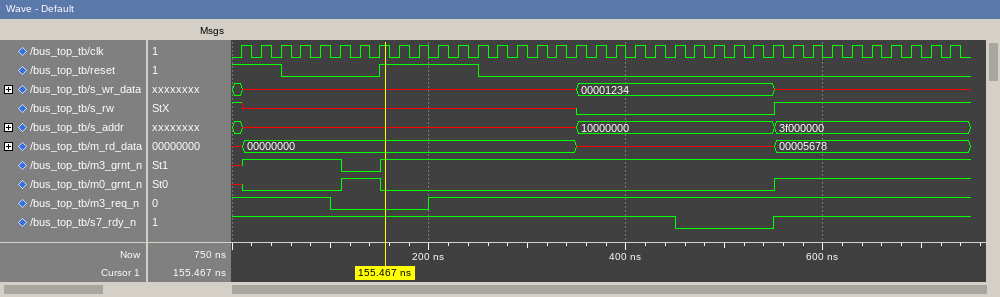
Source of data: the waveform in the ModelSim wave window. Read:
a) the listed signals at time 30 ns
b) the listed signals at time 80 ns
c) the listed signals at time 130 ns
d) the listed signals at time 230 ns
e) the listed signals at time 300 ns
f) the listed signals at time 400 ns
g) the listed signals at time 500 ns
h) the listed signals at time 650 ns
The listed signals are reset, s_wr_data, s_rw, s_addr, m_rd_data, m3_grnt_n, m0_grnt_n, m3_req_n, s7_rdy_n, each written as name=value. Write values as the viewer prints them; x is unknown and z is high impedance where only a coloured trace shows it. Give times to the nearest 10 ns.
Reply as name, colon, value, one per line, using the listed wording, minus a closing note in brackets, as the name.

the listed signals at time 30 ns: reset=1, s_wr_data=x, s_rw=x, s_addr=x, m_rd_data=00000000, m3_grnt_n=1, m0_grnt_n=0, m3_req_n=1, s7_rdy_n=1
the listed signals at time 80 ns: reset=0, s_wr_data=x, s_rw=x, s_addr=x, m_rd_data=00000000, m3_grnt_n=1, m0_grnt_n=0, m3_req_n=1, s7_rdy_n=1
the listed signals at time 130 ns: reset=0, s_wr_data=x, s_rw=x, s_addr=x, m_rd_data=00000000, m3_grnt_n=0, m0_grnt_n=1, m3_req_n=0, s7_rdy_n=1
the listed signals at time 230 ns: reset=1, s_wr_data=x, s_rw=x, s_addr=x, m_rd_data=00000000, m3_grnt_n=1, m0_grnt_n=0, m3_req_n=1, s7_rdy_n=1
the listed signals at time 300 ns: reset=0, s_wr_data=x, s_rw=x, s_addr=x, m_rd_data=00000000, m3_grnt_n=1, m0_grnt_n=0, m3_req_n=1, s7_rdy_n=1
the listed signals at time 400 ns: reset=0, s_wr_data=00001234, s_rw=0, s_addr=10000000, m_rd_data=x, m3_grnt_n=1, m0_grnt_n=0, m3_req_n=1, s7_rdy_n=1
the listed signals at time 500 ns: reset=0, s_wr_data=00001234, s_rw=0, s_addr=10000000, m_rd_data=x, m3_grnt_n=1, m0_grnt_n=0, m3_req_n=1, s7_rdy_n=0
the listed signals at time 650 ns: reset=0, s_wr_data=x, s_rw=1, s_addr=3f000000, m_rd_data=00005678, m3_grnt_n=1, m0_grnt_n=1, m3_req_n=1, s7_rdy_n=1
